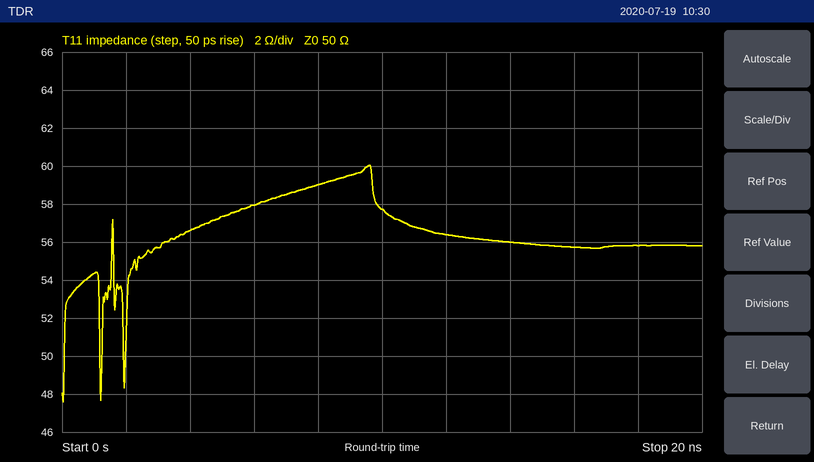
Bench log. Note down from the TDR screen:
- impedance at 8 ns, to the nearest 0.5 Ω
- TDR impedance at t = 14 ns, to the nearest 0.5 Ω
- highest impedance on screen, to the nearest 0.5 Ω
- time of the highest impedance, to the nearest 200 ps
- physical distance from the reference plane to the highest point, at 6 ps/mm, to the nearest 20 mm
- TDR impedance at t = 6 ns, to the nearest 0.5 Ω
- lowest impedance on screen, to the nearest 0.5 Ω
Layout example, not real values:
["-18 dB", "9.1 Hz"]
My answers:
["59.0 Ω", "56.0 Ω", "60.0 Ω", "9.6 ns", "800 mm", "58.0 Ω", "47.5 Ω"]
